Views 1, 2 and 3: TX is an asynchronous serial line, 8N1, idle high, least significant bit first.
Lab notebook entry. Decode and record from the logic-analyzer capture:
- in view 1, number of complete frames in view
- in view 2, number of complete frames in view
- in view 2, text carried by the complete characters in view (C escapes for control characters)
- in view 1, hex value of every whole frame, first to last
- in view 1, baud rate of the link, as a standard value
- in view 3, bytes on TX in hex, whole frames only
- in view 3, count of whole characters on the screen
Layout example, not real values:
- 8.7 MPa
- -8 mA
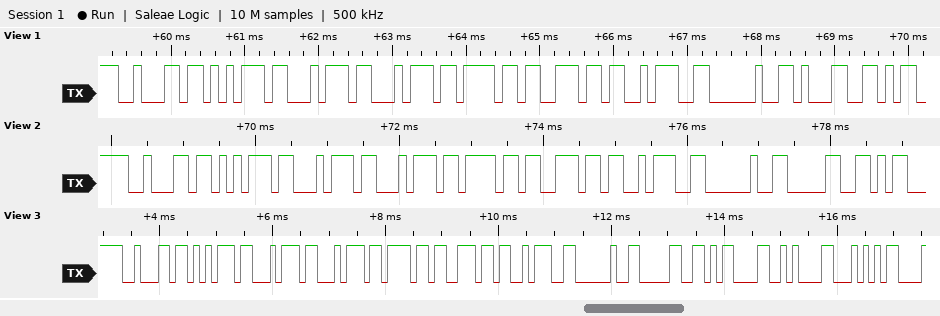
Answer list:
- 9
- 9
- "button: 0"
- 62 75 74 74 6F 6E 3A 20 31
- 9600 baud
- 62 75 74 74 6F 6E 3A 20 30 0D 0A 54
- 12
